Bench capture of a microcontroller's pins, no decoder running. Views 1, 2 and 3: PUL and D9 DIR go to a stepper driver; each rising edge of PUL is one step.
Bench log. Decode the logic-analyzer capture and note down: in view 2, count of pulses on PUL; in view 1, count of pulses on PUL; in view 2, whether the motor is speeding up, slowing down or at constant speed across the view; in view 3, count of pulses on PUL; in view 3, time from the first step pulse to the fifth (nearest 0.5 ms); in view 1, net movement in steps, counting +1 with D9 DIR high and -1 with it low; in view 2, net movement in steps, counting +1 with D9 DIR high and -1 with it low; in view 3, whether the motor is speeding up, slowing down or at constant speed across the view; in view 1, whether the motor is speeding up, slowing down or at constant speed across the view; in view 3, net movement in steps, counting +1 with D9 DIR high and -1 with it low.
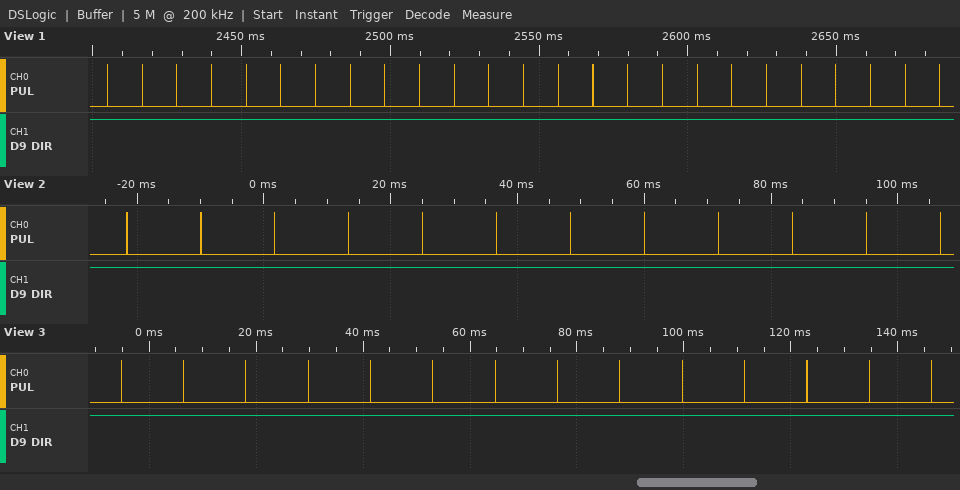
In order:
12
25
constant speed
14
46.5 ms
+25
+12
constant speed
constant speed
+14
